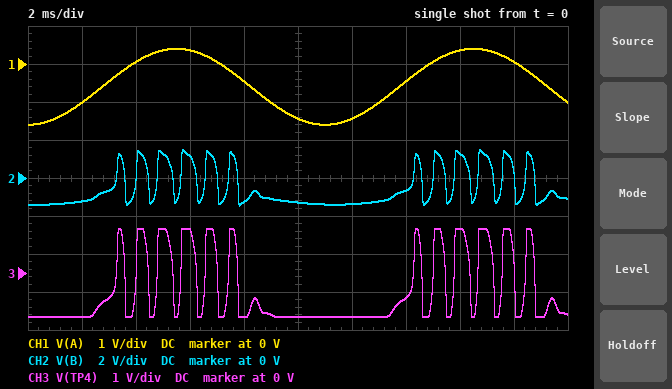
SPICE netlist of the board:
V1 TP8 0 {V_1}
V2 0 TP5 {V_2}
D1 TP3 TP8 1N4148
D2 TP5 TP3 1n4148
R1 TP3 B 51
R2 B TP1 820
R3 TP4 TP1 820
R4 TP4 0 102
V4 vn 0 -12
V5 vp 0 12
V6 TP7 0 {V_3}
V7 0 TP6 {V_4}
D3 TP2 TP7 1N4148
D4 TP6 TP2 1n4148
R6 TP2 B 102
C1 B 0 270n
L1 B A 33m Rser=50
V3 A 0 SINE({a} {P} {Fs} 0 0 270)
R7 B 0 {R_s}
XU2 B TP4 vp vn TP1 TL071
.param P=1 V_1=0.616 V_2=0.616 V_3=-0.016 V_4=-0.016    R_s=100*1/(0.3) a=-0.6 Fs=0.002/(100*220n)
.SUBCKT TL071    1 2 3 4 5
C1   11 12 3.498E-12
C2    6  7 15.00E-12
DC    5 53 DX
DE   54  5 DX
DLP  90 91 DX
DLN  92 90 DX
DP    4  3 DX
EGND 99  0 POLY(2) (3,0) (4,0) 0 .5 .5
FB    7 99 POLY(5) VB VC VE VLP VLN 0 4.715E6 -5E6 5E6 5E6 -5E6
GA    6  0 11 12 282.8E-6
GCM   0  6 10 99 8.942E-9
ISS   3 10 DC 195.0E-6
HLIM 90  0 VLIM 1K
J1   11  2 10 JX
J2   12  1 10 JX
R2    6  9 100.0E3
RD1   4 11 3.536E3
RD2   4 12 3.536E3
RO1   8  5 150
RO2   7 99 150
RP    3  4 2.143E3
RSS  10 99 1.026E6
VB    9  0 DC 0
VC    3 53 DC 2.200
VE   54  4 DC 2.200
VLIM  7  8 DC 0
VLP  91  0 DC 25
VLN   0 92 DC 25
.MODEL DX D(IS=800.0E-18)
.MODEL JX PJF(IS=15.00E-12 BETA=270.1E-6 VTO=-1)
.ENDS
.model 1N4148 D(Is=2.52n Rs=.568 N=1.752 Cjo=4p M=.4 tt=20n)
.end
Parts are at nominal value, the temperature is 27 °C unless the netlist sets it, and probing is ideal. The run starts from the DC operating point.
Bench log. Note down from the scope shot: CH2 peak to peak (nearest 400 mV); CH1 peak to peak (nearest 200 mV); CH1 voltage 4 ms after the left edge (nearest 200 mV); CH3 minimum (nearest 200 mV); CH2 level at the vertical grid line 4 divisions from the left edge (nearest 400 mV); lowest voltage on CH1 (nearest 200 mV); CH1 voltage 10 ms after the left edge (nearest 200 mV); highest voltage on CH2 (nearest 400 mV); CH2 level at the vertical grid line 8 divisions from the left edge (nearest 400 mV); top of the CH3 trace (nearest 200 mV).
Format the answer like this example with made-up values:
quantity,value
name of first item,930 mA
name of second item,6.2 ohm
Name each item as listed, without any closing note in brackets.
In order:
quantity,value
CH2 peak to peak,2.8 V
CH1 peak to peak,2.0 V
CH1 voltage 4 ms after the left edge,0 V
CH3 minimum,-1.2 V
CH2 level at the vertical grid line 4 divisions from the left edge,-1.2 V
lowest voltage on CH1,-1.6 V
CH1 voltage 10 ms after the left edge,-1.4 V
highest voltage on CH2,1.6 V
CH2 level at the vertical grid line 8 divisions from the left edge,1.2 V
top of the CH3 trace,1.2 V
